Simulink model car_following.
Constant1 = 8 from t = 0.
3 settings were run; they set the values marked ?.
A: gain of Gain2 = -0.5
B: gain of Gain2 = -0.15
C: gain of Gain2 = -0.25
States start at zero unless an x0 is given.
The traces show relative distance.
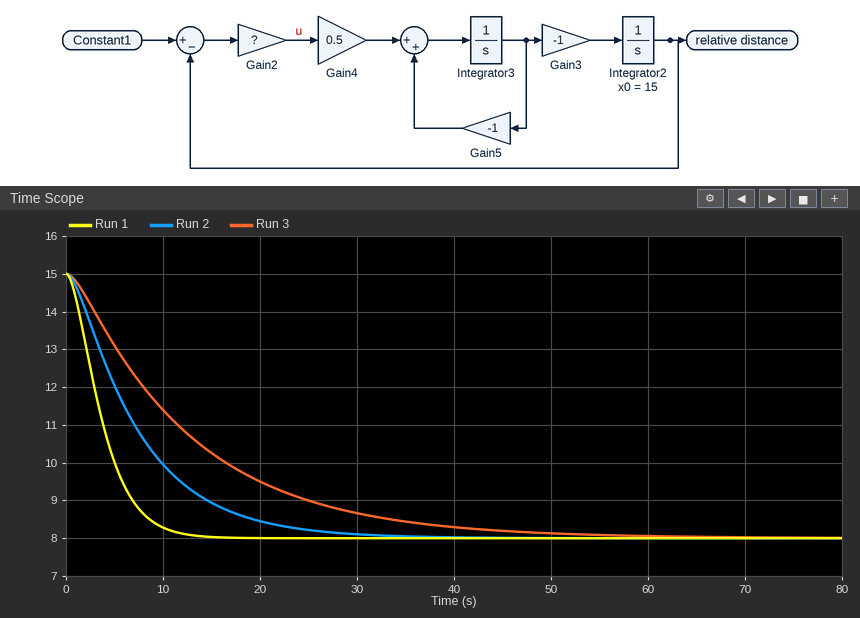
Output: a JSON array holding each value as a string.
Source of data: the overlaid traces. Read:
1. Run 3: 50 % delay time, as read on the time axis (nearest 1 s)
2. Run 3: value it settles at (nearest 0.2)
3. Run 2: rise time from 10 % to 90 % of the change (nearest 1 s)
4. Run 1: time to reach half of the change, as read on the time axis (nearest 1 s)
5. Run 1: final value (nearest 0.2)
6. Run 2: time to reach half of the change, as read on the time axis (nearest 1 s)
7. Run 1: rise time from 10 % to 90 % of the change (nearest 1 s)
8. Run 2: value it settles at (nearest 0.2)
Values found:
["10 s", "8.0", "15 s", "3 s", "8.0", "6 s", "7 s", "8.0"]
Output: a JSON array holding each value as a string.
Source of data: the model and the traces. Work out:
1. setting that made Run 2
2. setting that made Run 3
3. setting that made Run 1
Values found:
["C", "B", "A"]
